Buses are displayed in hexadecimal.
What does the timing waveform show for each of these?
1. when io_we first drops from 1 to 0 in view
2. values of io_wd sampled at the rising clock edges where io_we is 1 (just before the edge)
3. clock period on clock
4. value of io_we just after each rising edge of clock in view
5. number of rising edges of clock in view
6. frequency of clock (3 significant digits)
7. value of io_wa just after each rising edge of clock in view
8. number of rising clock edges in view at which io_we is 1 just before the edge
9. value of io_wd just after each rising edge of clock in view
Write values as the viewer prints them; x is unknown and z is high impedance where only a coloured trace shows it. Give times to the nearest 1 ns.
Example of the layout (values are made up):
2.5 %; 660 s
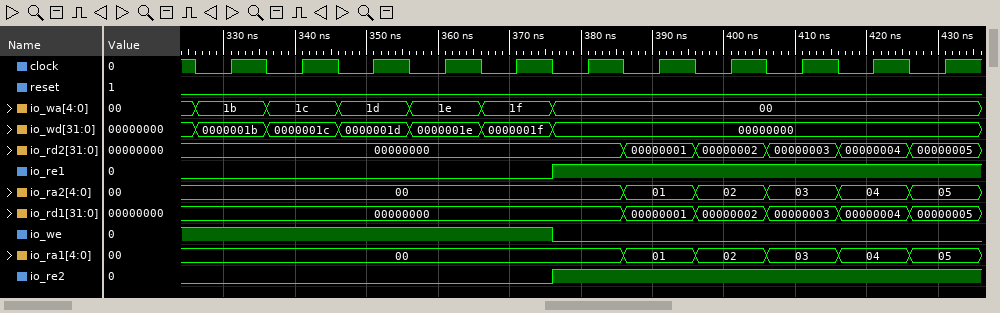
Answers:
376 ns; 0000001b, 0000001c, 0000001d, 0000001e, 0000001f; 10 ns; 1 1 1 1 1 0 0 0 0 0 0; 11; 100 MHz; 1b, 1c, 1d, 1e, 1f, 00, 00, 00, 00, 00, 00; 5; 0000001b, 0000001c, 0000001d, 0000001e, 0000001f, 00000000, 00000000, 00000000, 00000000, 00000000, 00000000
